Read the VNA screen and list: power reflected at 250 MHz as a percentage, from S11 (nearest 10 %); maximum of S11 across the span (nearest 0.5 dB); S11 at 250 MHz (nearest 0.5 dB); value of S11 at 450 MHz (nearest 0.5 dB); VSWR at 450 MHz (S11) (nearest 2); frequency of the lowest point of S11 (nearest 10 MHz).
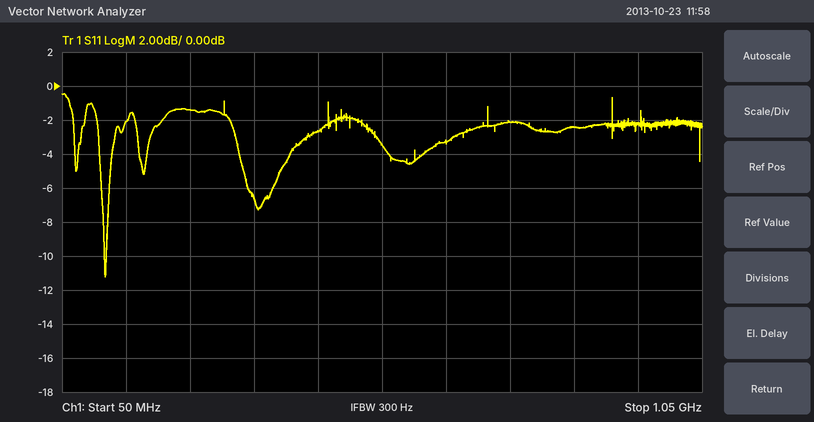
70 %
-0.5 dB
-1.5 dB
-2.5 dB
6
120 MHz
